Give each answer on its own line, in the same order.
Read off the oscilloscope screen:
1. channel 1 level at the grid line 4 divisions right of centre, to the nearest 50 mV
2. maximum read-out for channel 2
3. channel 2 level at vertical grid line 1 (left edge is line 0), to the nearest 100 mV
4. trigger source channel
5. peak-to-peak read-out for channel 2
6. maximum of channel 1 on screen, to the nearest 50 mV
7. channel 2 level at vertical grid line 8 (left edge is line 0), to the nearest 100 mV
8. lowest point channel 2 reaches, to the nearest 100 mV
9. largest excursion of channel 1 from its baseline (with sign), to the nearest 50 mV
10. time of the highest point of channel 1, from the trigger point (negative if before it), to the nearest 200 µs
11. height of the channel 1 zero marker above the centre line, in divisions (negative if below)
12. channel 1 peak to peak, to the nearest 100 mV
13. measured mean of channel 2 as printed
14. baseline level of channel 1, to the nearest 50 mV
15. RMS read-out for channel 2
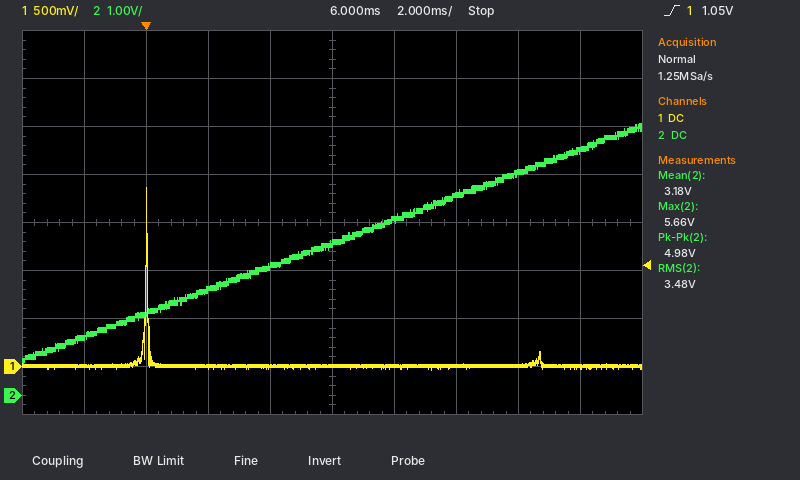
0 mV
5.66 V
1.2 V
channel 1
4.98 V
1.85 V
4.6 V
700 mV
+1.85 V
0.0 ms
-3.0 div
1.90 V
3.18 V
0 mV
3.48 V
